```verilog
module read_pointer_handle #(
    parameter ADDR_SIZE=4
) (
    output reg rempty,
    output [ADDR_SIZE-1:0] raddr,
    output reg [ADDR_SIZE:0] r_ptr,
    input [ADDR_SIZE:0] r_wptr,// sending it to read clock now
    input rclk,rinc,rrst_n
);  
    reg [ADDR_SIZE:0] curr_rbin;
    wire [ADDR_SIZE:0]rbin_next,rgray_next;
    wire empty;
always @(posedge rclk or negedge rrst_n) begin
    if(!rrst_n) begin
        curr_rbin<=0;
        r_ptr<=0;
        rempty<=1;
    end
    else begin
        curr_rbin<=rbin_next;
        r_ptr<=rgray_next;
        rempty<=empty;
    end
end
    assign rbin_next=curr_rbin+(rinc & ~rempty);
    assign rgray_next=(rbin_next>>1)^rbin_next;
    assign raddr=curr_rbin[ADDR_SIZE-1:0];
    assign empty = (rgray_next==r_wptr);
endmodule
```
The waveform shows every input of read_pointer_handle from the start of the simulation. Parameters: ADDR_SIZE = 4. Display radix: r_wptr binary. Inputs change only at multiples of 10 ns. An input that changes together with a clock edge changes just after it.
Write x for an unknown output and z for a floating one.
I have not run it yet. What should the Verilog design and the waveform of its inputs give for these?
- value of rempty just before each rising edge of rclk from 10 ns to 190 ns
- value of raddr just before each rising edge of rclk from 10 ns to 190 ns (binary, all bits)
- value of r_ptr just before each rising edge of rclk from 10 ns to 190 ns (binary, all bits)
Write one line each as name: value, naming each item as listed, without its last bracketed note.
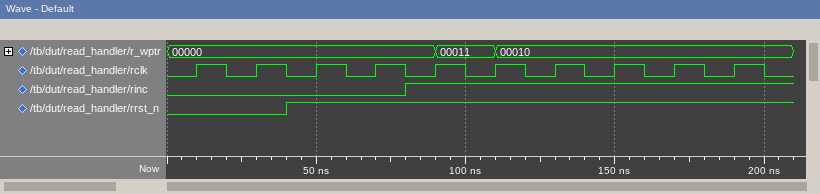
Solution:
value of rempty just before each rising edge of rclk from 10 ns to 190 ns: 1 1 1 1 1 1 0 0 0 1
value of raddr just before each rising edge of rclk from 10 ns to 190 ns: 0000, 0000, 0000, 0000, 0000, 0000, 0000, 0001, 0010, 0011
value of r_ptr just before each rising edge of rclk from 10 ns to 190 ns: 00000, 00000, 00000, 00000, 00000, 00000, 00000, 00001, 00011, 00010
